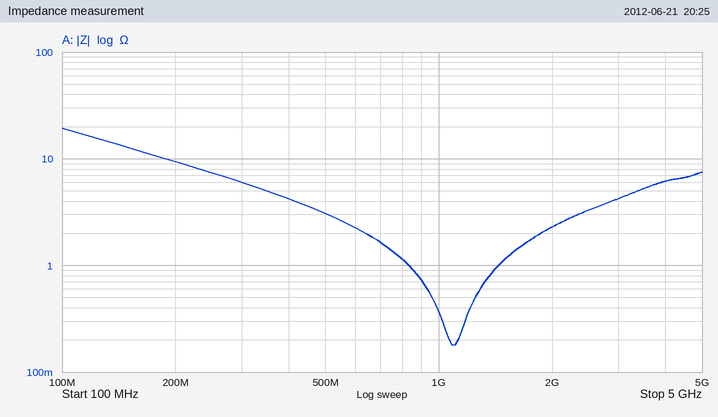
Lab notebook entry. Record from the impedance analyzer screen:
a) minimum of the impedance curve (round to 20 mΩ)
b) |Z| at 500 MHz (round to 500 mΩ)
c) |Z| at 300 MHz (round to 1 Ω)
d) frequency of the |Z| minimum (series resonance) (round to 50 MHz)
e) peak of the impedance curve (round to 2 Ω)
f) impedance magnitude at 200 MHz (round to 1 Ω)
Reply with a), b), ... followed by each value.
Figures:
a) 180 mΩ
b) 3.0 Ω
c) 6 Ω
d) 1.10 GHz
e) 20 Ω
f) 9 Ω
